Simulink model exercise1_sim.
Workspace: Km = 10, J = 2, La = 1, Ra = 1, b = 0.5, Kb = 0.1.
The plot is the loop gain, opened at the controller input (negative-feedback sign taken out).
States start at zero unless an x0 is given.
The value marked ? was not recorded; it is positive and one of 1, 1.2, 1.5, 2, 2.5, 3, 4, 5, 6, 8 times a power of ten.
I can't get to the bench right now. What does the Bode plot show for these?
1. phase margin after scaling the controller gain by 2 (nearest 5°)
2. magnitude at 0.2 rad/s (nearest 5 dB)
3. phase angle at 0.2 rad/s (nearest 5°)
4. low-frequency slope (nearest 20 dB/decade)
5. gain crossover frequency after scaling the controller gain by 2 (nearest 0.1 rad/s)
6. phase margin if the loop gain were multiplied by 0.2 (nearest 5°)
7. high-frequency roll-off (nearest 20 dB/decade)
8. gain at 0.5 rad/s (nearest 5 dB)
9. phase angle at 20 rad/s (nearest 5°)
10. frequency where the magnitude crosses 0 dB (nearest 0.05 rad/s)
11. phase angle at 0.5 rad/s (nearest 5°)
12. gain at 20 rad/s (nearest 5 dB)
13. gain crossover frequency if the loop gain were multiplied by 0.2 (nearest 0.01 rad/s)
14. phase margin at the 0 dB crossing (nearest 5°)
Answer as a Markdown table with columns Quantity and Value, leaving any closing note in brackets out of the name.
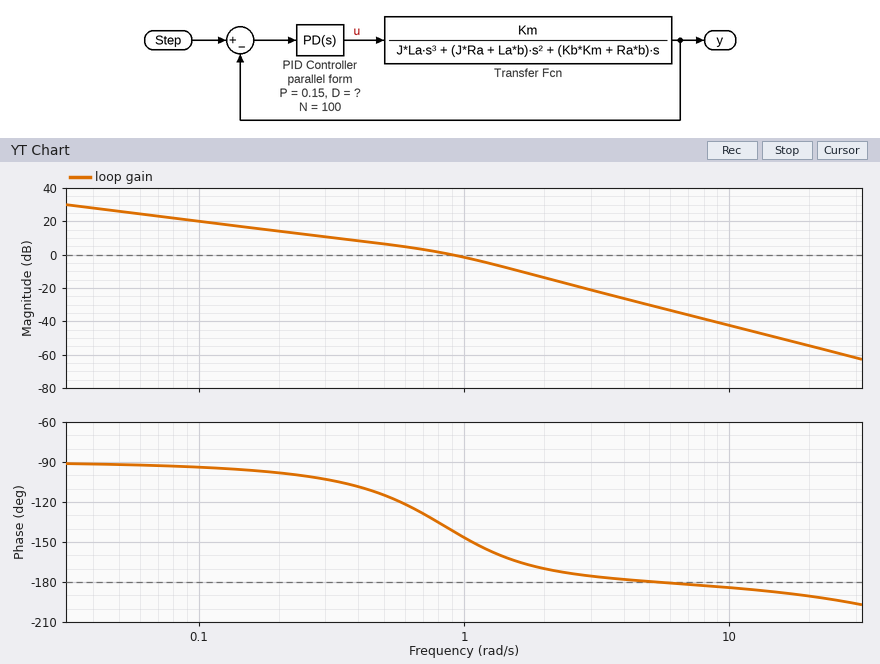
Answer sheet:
| Quantity | Value |
|---|---|
| phase margin after scaling the controller gain by 2 | 20° |
| magnitude at 0.2 rad/s | 15 dB |
| phase angle at 0.2 rad/s | -100° |
| low-frequency slope | -20 dB/decade |
| gain crossover frequency after scaling the controller gain by 2 | 1.3 rad/s |
| phase margin if the loop gain were multiplied by 0.2 | 80° |
| high-frequency roll-off | -40 dB/decade |
| gain at 0.5 rad/s | 5 dB |
| phase angle at 20 rad/s | -190° |
| frequency where the magnitude crosses 0 dB | 0.90 rad/s |
| phase angle at 0.5 rad/s | -115° |
| gain at 20 rad/s | -55 dB |
| gain crossover frequency if the loop gain were multiplied by 0.2 | 0.20 rad/s |
| phase margin at the 0 dB crossing | 40° |
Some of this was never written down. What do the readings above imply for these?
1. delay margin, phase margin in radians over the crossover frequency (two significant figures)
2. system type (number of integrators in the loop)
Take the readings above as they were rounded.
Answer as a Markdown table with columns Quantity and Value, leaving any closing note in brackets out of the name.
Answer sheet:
| Quantity | Value |
|---|---|
| delay margin, phase margin in radians over the crossover frequency | 0.78 s |
| system type | 1 |
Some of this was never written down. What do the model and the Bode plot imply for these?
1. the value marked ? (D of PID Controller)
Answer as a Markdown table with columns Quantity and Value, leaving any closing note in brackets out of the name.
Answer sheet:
| Quantity | Value |
|---|---|
| the value marked ? | 0.15 |
